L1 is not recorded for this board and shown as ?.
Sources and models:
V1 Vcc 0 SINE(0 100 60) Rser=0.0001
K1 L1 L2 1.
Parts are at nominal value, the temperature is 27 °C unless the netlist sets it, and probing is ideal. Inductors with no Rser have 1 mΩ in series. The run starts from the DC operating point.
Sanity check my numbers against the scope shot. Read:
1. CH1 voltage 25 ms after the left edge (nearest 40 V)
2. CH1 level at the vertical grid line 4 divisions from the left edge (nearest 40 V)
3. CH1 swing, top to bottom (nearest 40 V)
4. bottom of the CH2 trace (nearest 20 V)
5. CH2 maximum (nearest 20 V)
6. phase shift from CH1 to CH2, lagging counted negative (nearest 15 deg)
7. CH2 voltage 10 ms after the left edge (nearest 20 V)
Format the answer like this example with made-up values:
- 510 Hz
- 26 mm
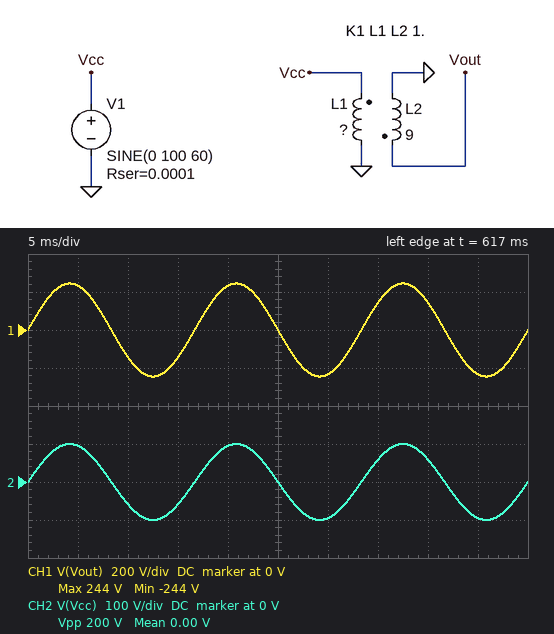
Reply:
- 0 V
- 240 V
- 480 V
- -100 V
- 100 V
- 0 deg
- -60 V
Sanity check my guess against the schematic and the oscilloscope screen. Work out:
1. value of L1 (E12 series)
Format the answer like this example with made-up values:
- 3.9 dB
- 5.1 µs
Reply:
- 1.5 H
